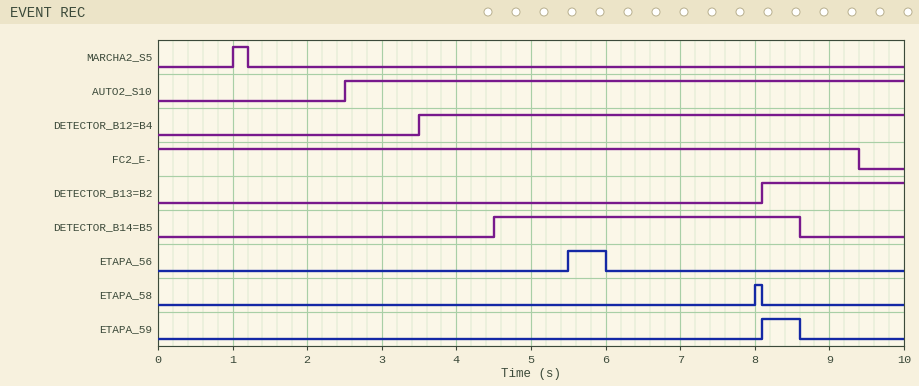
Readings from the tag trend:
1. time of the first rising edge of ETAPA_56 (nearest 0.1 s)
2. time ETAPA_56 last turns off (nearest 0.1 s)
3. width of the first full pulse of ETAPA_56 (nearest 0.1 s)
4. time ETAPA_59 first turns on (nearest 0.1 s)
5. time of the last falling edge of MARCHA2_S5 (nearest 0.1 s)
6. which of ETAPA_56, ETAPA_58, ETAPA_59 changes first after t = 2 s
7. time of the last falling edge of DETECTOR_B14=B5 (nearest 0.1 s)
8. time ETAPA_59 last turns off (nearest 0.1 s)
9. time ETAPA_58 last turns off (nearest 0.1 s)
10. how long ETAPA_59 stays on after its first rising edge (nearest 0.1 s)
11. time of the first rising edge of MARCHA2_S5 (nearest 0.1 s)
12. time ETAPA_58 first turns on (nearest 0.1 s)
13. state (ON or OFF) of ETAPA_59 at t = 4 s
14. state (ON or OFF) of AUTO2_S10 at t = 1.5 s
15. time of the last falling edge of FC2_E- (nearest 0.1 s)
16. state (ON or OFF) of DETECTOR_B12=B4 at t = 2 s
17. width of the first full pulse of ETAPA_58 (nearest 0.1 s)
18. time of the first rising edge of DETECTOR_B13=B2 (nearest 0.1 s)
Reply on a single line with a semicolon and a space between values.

5.5 s; 6.0 s; 0.5 s; 8.1 s; 1.2 s; ETAPA_56; 8.6 s; 8.6 s; 8.1 s; 0.5 s; 1.0 s; 8.0 s; OFF; OFF; 9.4 s; OFF; 0.1 s; 8.1 s
